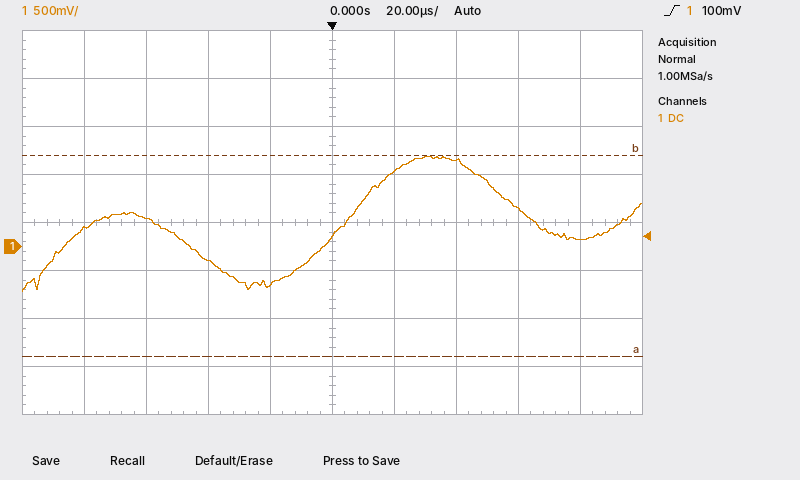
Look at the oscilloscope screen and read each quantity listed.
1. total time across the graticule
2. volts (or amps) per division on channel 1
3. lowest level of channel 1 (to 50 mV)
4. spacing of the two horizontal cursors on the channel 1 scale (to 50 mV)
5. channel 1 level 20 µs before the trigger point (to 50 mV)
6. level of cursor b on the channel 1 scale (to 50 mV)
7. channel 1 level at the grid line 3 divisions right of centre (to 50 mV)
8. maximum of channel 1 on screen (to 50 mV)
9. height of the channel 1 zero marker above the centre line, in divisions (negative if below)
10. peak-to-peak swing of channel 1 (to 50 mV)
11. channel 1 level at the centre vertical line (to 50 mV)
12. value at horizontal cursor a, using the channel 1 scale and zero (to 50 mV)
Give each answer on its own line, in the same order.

200 µs
500 mV
-450 mV
2.10 V
-400 mV
950 mV
400 mV
950 mV
-0.5 div
1.40 V
100 mV
-1.15 V
